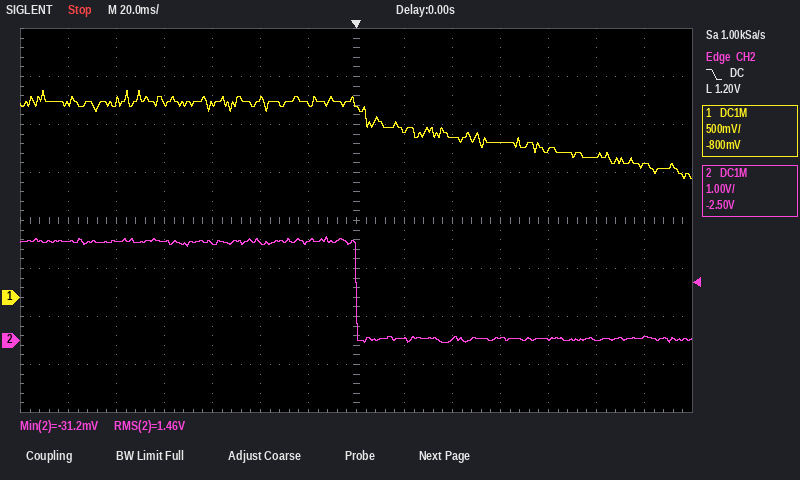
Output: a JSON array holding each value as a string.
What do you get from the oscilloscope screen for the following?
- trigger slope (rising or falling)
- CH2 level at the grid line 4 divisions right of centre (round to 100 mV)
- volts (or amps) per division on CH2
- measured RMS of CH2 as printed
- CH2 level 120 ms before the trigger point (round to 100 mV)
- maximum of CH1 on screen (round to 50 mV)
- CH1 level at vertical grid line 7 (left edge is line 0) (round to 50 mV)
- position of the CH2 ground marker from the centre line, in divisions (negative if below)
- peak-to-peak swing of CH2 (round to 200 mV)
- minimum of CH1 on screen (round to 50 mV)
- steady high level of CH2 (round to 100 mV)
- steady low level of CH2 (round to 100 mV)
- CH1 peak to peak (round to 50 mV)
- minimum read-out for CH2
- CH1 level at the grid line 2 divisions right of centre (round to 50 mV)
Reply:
["falling", "0.0 V", "1 V", "1.46 V", "2.1 V", "2.15 V", "2.00 V", "-2.5 div", "2.2 V", "1.25 V", "2.1 V", "0.0 V", "900 mV", "-31.2 mV", "1.65 V"]
